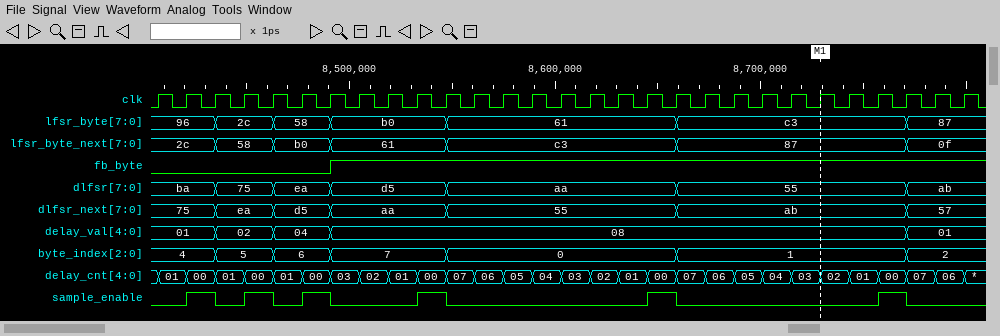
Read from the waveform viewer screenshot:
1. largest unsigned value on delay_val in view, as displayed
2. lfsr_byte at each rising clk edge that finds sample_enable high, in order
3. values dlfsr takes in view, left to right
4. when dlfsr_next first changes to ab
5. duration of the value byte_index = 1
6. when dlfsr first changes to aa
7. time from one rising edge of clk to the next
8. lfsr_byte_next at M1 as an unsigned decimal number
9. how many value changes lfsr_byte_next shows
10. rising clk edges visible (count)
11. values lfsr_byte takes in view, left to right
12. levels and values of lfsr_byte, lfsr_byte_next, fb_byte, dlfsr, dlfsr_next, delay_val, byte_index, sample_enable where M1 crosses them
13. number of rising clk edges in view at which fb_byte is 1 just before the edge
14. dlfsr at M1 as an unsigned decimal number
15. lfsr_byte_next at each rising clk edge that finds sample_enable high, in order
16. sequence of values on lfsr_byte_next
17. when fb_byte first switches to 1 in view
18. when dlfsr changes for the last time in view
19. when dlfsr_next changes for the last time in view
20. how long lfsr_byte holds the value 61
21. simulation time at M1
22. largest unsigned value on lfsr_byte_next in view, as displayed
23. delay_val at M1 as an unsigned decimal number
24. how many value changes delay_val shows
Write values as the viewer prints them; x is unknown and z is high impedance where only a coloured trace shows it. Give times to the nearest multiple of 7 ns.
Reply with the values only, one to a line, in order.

08
96, 2c, 58, b0, 61, c3
ba, 75, ea, d5, aa, 55, ab
8659 ns
112 ns
8547 ns
14 ns
135
6
29
96, 2c, 58, b0, 61, c3, 87
lfsr_byte=c3, lfsr_byte_next=87, fb_byte=1, dlfsr=55, dlfsr_next=ab, delay_val=08, byte_index=1, sample_enable=0
22
85
2c, 58, b0, 61, c3, 87
2c, 58, b0, 61, c3, 87, 0f
8491 ns
8771 ns
8771 ns
112 ns
8729 ns
c3
8
4
